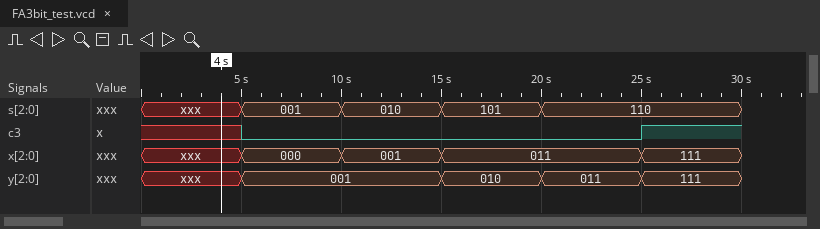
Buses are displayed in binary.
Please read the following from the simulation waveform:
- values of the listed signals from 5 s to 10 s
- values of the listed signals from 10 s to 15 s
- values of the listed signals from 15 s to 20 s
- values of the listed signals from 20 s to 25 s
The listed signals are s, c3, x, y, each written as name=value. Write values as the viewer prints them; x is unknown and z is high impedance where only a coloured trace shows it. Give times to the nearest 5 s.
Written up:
s=001, c3=0, x=000, y=001
s=010, c3=0, x=001, y=001
s=101, c3=0, x=011, y=010
s=110, c3=0, x=011, y=011
